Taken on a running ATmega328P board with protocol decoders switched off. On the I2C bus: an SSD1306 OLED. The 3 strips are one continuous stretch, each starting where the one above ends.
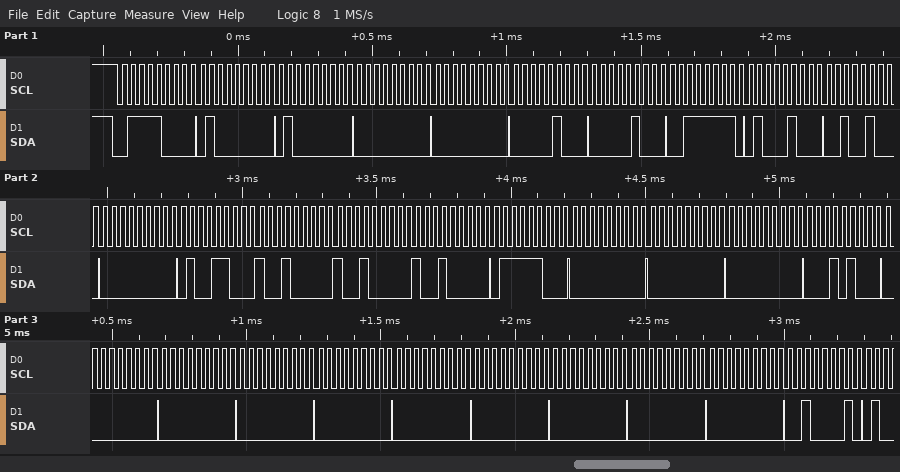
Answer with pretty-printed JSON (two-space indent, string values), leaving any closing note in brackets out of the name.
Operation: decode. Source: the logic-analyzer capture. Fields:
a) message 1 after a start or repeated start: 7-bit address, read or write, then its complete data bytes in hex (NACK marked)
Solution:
{
  "message 1 after a start or repeated start: 7-bit address, read or write, then its complete data bytes in hex": "0x3C write: 40 40 00 00 04 04 3F 44 24 00 4C 90 90 90 7C 00 00 00 14 00 00 00 00 00 00 00 00 00 21"
}
